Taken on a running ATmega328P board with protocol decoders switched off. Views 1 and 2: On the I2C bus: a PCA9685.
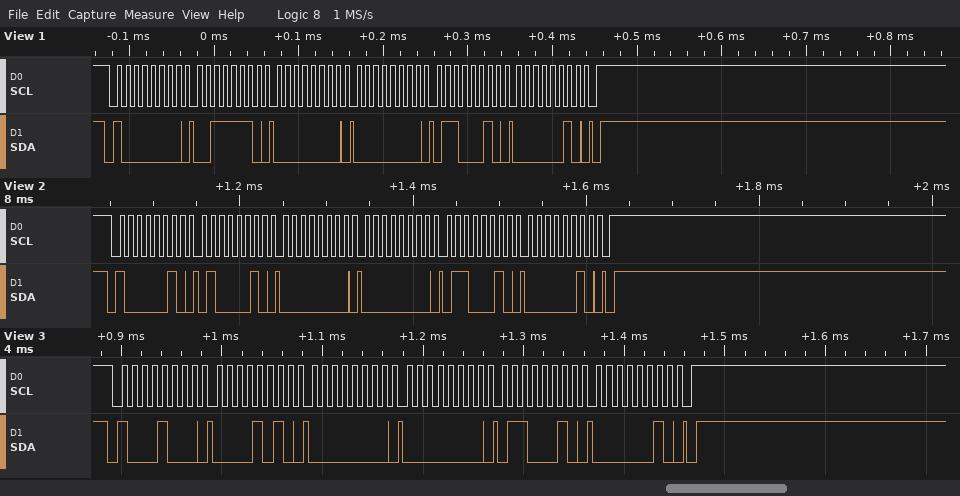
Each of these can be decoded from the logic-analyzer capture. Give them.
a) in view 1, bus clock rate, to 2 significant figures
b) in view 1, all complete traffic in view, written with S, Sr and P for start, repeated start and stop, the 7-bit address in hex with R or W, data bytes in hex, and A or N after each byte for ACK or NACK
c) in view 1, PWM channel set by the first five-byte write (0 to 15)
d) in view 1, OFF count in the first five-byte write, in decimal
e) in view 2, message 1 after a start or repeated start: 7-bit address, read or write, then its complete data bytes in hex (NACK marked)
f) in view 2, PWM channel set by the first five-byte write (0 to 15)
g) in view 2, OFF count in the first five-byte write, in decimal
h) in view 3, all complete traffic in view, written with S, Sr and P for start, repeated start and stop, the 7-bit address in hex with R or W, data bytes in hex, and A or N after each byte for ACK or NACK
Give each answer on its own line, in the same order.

100 kHz
S 40W A 3E A 00 A 00 A 62 A 02 A P
14
610
0x41 write: 42 00 00 62 02
15
610
S 44W A 0A A 00 A 00 A 62 A 02 A P
